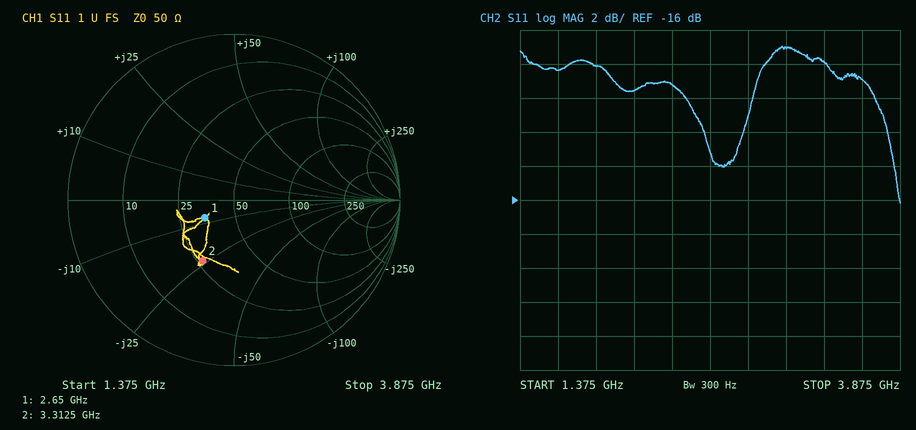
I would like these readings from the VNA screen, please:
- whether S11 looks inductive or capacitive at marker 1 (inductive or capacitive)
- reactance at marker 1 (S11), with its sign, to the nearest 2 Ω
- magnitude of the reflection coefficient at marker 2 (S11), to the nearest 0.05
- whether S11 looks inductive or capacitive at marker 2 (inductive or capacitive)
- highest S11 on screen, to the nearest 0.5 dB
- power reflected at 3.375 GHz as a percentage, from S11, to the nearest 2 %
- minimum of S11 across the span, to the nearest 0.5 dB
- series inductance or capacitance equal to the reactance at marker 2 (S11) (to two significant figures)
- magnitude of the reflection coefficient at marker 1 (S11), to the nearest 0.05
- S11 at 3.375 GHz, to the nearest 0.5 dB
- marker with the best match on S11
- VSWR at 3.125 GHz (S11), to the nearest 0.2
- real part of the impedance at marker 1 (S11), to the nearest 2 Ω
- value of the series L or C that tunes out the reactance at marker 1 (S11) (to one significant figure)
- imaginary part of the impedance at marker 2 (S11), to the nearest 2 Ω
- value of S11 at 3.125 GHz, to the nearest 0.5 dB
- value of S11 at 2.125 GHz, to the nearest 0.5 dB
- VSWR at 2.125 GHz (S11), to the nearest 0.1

capacitive
-8 Ω
0.40
capacitive
-7.0 dB
16 %
-16.0 dB
2.0 pF
0.20
-8.0 dB
marker 1
2.6
34 Ω
500 pH
-24 Ω
-7.0 dB
-9.5 dB
2.0
